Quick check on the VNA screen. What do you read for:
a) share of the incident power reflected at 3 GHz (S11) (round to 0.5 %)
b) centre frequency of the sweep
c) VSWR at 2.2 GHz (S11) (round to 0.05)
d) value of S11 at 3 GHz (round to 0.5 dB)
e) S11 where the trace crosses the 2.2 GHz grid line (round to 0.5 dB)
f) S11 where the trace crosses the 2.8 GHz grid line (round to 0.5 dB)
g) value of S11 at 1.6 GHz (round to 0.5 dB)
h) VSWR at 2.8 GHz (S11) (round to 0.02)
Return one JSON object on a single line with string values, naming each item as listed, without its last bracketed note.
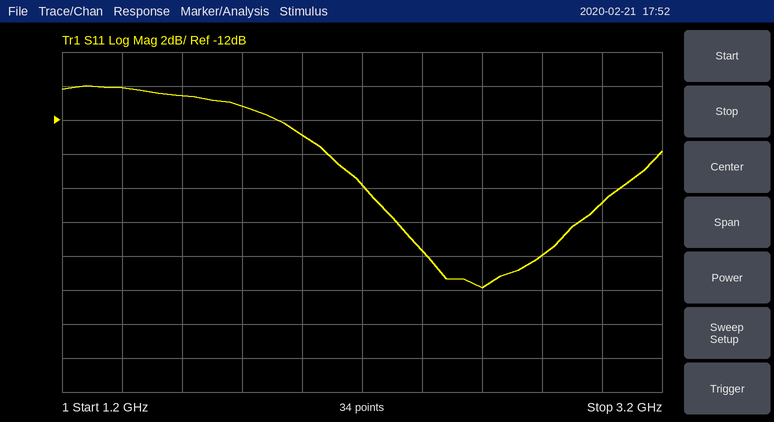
{"share of the incident power reflected at 3 GHz (S11)": "2.0 %", "centre frequency of the sweep": "2.2 GHz", "VSWR at 2.2 GHz (S11)": "1.40", "value of S11 at 3 GHz": "-17.0 dB", "S11 where the trace crosses the 2.2 GHz grid line": "-16.0 dB", "S11 where the trace crosses the 2.8 GHz grid line": "-20.0 dB", "value of S11 at 1.6 GHz": "-10.5 dB", "VSWR at 2.8 GHz (S11)": "1.22"}
